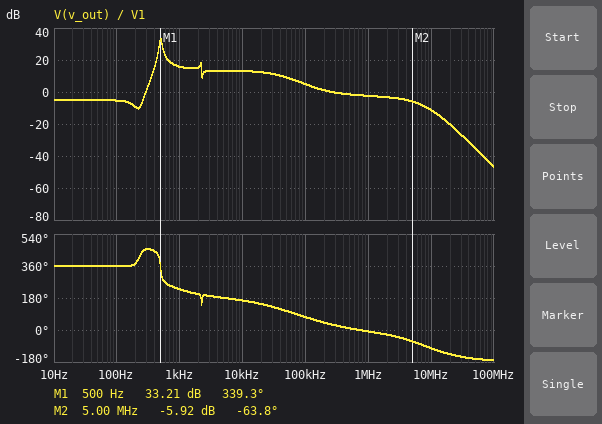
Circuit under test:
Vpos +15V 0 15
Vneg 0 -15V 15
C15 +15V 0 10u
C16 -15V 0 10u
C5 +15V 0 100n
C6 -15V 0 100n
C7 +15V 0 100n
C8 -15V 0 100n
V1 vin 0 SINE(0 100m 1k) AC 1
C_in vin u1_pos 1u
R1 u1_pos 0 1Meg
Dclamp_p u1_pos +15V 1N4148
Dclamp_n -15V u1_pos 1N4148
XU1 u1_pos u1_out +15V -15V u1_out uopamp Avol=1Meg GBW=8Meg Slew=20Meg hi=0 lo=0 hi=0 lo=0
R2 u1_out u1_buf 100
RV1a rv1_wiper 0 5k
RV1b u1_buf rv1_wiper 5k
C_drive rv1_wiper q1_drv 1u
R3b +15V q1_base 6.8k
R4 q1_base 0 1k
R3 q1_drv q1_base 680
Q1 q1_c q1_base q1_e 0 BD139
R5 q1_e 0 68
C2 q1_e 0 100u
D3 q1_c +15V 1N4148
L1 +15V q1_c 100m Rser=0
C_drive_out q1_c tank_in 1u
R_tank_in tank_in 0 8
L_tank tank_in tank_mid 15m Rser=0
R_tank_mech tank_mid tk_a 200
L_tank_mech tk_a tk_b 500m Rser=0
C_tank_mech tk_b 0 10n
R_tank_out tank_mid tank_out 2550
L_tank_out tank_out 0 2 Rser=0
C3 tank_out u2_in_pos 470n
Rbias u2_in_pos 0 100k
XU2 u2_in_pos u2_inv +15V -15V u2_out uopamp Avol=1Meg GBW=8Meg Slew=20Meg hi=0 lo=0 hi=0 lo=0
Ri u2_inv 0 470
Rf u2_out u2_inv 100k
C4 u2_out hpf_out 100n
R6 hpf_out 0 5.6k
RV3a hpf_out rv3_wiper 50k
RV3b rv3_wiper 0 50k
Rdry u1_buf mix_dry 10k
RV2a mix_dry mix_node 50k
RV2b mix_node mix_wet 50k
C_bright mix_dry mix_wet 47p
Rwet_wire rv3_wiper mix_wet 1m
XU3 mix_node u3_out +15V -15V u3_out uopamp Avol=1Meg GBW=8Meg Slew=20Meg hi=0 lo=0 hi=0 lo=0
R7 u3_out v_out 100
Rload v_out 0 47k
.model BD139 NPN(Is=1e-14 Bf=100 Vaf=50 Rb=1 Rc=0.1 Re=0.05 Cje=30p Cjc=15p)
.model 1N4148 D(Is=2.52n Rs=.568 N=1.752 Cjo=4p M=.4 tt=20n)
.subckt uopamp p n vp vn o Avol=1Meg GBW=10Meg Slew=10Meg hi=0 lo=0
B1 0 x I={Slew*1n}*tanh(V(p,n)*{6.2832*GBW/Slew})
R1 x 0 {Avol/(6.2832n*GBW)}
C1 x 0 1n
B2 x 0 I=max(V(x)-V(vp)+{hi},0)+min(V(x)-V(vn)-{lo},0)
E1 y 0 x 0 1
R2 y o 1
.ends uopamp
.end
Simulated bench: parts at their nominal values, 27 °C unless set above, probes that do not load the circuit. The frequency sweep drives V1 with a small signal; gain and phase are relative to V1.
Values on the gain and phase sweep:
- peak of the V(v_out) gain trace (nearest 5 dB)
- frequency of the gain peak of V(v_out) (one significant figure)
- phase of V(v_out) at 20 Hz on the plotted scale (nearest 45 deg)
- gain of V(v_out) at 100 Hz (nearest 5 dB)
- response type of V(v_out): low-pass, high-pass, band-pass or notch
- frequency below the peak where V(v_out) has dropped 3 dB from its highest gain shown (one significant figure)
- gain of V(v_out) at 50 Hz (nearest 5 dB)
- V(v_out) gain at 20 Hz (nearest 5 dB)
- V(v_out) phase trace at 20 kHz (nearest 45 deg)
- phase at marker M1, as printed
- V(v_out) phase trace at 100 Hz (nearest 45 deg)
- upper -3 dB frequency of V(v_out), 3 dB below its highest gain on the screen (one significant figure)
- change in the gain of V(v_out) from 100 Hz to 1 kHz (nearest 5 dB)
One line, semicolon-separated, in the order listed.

35 dB; 500 Hz; 360 deg; -5 dB; band-pass; 500 Hz; -5 dB; -5 dB; 135 deg; 339.3 deg; 360 deg; 500 Hz; 20 dB
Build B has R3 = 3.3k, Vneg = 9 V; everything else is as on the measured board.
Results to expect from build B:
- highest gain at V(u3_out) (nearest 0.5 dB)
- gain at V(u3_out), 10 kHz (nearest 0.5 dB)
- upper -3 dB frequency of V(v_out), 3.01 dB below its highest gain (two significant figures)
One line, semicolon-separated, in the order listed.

28.0 dB; 7.5 dB; 520 Hz
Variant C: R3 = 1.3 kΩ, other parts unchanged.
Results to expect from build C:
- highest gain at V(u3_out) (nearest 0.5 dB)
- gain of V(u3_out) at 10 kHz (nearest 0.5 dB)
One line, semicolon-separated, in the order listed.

32.0 dB; 11.5 dB
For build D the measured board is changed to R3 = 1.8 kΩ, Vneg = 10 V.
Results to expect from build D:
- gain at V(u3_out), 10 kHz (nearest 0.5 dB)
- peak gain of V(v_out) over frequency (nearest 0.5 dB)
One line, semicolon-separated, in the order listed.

10.5 dB; 30.5 dB
